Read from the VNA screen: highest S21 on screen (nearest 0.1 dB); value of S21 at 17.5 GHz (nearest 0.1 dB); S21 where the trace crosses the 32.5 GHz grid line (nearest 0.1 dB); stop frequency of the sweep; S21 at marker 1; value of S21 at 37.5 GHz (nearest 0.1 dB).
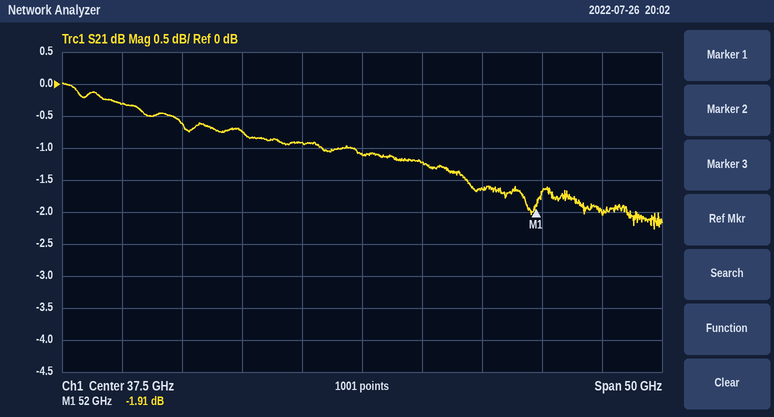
0.0 dB
-0.3 dB
-0.9 dB
62.5 GHz
-1.91 dB
-1.1 dB
